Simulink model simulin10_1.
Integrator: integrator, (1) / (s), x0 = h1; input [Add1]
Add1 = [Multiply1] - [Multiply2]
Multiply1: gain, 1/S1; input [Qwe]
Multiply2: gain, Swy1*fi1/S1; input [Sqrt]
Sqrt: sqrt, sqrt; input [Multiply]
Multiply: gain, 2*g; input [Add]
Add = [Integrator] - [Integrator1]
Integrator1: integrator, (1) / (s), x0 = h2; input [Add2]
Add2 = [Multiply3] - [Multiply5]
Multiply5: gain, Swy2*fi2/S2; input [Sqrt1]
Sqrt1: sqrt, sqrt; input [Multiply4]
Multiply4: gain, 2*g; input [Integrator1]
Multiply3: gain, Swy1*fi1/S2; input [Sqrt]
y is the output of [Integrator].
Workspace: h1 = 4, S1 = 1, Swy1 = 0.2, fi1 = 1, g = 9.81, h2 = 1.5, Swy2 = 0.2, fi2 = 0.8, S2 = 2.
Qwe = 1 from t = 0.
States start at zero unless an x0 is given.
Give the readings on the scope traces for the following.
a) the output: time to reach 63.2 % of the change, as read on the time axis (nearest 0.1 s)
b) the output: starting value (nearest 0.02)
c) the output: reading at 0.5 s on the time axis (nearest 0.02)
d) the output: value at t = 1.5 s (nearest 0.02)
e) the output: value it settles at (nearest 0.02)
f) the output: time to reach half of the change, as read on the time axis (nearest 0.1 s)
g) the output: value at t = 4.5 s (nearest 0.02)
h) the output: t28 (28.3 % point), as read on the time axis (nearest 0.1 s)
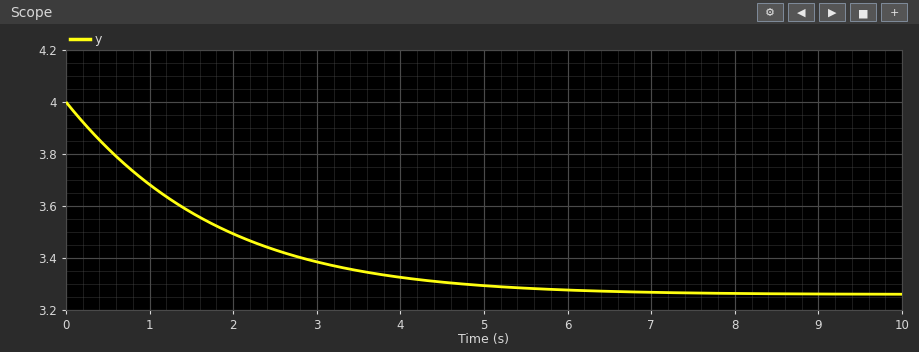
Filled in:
1.7 s
4.00
3.82
3.58
3.26
1.2 s
3.30
0.6 s
